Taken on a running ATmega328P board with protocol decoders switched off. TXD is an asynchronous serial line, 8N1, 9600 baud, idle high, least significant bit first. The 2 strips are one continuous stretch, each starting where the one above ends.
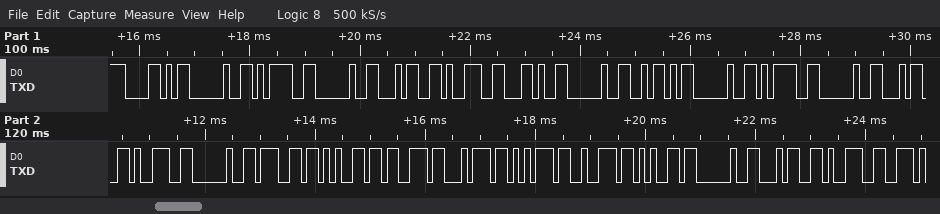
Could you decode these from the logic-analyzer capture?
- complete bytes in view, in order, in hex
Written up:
0x58 0x20 0x3D 0x20 0x34 0x39 0x2C 0x20 0x5A 0x20 0x3D 0x20 0x34 0x39 0x20 0x67 0x65 0x73 0x74 0x75 0x72 0x65 0x20 0x34 0x39
